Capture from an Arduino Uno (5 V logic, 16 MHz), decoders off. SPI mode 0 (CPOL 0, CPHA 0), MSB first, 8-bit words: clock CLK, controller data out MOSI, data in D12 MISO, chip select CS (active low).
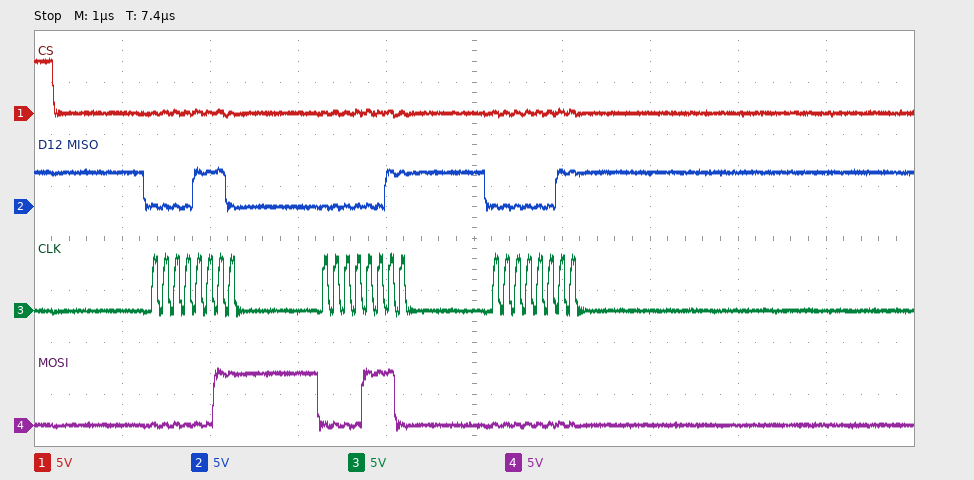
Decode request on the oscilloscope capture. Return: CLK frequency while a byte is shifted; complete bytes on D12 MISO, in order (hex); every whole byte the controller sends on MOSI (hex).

8 MHz
0E 03 03
03 0E 00
